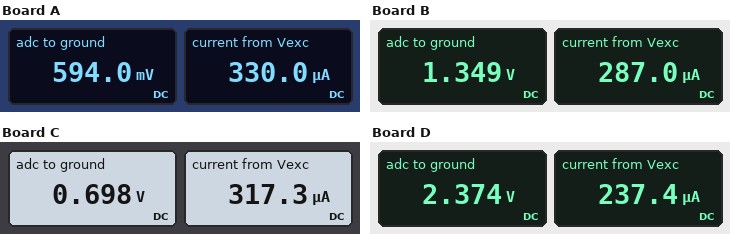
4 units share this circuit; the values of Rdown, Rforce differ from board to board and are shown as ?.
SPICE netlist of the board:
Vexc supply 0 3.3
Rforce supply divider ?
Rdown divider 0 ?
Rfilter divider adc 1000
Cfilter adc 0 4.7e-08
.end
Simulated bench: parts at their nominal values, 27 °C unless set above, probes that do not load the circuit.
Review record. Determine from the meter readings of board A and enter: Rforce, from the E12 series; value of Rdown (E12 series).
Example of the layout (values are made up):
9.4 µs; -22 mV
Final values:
8.2 kΩ; 1.8 kΩ
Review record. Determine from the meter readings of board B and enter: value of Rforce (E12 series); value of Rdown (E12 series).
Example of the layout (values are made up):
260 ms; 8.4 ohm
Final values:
6.8 kΩ; 4.7 kΩ
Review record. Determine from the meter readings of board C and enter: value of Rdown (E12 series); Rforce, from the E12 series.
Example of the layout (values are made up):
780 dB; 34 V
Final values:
2.2 kΩ; 8.2 kΩ
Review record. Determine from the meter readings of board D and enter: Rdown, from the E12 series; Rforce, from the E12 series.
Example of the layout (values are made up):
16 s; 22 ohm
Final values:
10 kΩ; 3.9 kΩ
